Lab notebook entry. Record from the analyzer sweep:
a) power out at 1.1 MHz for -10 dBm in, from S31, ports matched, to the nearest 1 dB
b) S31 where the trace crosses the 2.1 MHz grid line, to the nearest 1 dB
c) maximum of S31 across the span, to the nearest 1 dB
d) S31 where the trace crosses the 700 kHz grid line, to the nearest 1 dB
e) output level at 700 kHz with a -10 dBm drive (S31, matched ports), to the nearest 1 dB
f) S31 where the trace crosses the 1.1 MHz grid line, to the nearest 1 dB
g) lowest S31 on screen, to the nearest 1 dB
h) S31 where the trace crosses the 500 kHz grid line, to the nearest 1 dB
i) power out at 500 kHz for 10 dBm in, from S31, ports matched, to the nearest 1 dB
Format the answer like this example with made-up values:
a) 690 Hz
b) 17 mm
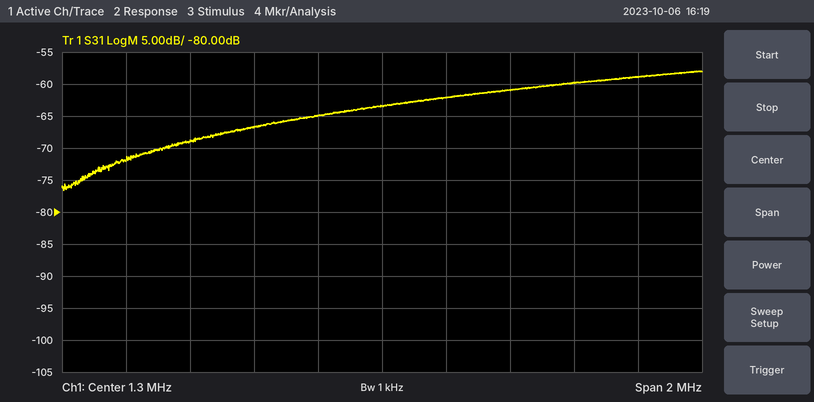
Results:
a) -75 dBm
b) -59 dB
c) -58 dB
d) -69 dB
e) -79 dBm
f) -65 dB
g) -77 dB
h) -72 dB
i) -62 dBm
